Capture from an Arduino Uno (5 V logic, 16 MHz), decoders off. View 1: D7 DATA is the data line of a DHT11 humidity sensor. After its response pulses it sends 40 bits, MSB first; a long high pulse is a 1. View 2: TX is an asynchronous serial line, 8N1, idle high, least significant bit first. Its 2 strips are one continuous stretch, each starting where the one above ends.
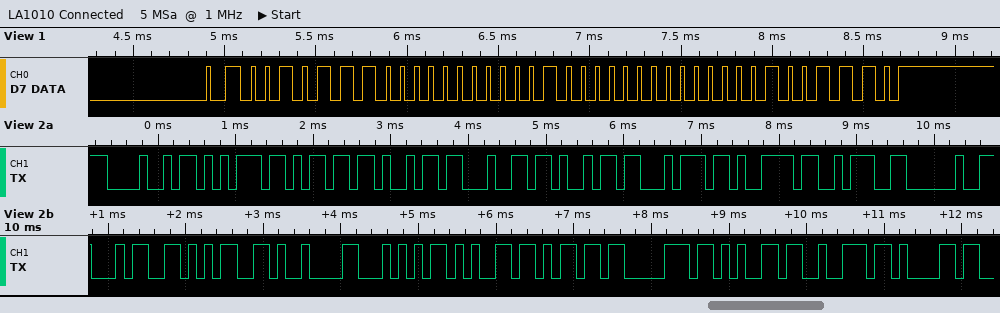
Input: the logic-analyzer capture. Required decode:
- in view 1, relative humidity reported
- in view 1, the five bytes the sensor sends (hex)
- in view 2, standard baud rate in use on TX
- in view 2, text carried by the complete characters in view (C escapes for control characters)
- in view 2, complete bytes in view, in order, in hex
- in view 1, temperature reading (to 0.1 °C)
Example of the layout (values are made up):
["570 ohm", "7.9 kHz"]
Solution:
["46 %", "2E 00 20 00 4E", "9600 baud", "\"Humidity: 45\\tTempera\"", "0x48 0x75 0x6D 0x69 0x64 0x69 0x74 0x79 0x3A 0x20 0x34 0x35 0x09 0x54 0x65 0x6D 0x70 0x65 0x72 0x61", "32.0 °C"]
